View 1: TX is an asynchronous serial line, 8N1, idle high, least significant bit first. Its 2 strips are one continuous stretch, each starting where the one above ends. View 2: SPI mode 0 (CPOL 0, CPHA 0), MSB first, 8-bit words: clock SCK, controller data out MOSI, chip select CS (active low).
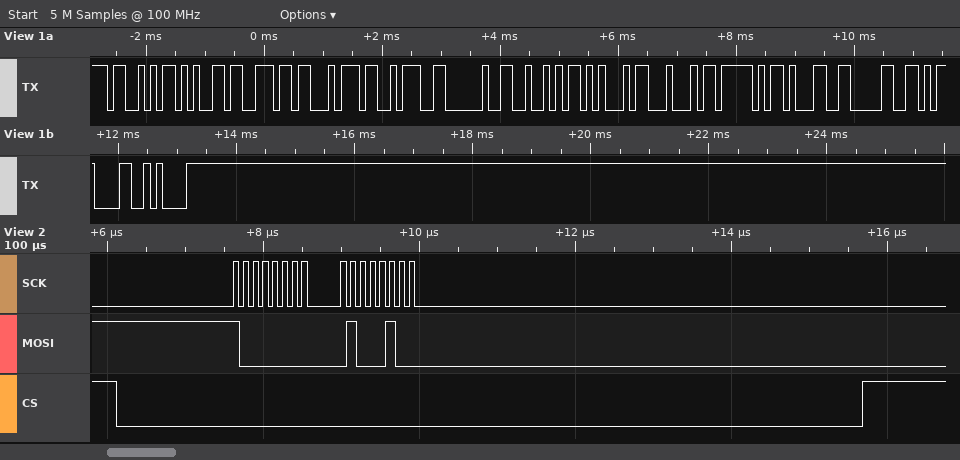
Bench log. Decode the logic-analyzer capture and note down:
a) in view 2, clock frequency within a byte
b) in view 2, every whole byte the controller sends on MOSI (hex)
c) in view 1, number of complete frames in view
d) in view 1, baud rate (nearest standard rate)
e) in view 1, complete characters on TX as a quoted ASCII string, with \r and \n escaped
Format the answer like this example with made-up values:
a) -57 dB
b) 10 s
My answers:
a) 8 MHz
b) 80 44
c) 14
d) 9600 baud
e) "Sent: RED_10\r\n"
